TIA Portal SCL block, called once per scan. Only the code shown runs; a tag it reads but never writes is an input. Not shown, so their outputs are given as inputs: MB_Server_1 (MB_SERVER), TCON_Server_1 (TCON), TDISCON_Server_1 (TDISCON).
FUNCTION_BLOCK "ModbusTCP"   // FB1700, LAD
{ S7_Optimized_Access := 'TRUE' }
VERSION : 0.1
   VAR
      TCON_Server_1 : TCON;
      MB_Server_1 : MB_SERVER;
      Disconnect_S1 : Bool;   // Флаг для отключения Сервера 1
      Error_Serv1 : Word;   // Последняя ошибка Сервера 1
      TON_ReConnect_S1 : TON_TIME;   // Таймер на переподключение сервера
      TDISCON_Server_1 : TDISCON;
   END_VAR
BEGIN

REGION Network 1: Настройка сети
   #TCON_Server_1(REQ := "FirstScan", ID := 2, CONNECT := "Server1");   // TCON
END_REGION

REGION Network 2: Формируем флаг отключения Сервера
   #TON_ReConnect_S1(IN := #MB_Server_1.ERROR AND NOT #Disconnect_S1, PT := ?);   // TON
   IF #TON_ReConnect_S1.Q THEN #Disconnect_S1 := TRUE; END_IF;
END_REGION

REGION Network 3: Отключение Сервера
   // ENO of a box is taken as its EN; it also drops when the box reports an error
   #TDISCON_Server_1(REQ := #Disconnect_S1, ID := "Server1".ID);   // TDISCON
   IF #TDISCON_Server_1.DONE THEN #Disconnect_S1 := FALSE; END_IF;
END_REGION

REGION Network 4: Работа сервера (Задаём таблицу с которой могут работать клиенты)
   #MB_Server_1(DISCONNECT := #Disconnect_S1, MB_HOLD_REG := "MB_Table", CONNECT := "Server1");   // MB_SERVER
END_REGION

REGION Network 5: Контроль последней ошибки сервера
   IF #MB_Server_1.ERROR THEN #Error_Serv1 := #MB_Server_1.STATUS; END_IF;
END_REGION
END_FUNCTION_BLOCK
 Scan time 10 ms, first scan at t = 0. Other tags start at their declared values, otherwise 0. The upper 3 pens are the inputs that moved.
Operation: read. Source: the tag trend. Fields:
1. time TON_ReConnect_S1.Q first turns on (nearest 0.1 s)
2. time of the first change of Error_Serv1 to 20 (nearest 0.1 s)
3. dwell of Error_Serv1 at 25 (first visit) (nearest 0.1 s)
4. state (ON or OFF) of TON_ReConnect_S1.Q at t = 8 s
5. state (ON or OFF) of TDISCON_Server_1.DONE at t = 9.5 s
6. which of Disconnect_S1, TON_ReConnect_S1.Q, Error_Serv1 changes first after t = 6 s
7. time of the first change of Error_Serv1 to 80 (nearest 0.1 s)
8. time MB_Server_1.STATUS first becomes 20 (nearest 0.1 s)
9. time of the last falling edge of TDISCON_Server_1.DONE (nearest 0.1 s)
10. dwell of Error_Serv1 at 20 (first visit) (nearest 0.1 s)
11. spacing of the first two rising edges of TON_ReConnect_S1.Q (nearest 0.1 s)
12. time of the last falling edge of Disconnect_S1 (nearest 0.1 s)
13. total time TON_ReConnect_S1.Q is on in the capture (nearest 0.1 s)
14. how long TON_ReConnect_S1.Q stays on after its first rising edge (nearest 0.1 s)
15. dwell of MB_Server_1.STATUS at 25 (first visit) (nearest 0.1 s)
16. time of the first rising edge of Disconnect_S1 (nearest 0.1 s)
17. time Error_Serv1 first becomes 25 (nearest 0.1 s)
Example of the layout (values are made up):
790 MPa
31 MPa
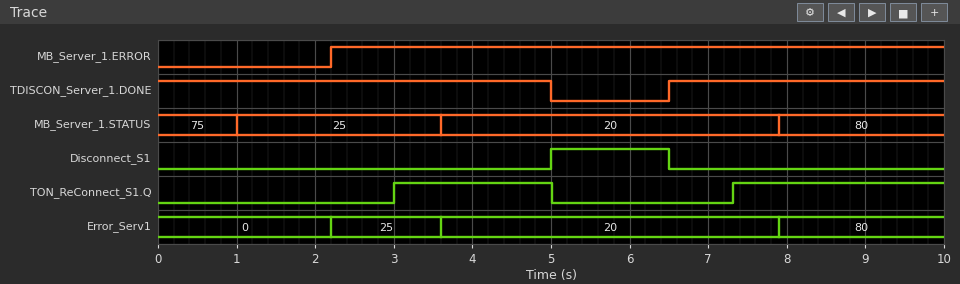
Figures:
3.0 s
3.6 s
1.4 s
ON
ON
Disconnect_S1
7.9 s
3.6 s
5.0 s
4.3 s
4.3 s
6.5 s
4.7 s
2.0 s
2.6 s
5.0 s
2.2 s
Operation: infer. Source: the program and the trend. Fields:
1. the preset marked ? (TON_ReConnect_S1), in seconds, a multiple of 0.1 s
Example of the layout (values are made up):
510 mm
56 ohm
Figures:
0.8 s
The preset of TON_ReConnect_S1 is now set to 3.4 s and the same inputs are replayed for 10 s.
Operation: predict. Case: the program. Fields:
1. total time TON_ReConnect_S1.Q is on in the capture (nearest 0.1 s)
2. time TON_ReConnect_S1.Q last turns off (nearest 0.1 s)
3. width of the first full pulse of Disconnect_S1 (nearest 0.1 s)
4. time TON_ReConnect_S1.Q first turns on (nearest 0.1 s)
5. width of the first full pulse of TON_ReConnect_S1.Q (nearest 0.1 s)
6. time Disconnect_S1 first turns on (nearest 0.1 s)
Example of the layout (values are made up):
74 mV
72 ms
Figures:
0.1 s
5.6 s
0.9 s
5.6 s
0.0 s
5.6 s
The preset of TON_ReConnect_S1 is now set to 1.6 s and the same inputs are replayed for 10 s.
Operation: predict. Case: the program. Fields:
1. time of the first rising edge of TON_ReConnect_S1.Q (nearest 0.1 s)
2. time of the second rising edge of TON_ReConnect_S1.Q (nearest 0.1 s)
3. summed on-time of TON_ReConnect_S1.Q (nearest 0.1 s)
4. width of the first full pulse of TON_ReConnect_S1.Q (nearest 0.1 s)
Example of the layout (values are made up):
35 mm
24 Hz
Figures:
3.8 s
8.1 s
3.1 s
1.2 s
